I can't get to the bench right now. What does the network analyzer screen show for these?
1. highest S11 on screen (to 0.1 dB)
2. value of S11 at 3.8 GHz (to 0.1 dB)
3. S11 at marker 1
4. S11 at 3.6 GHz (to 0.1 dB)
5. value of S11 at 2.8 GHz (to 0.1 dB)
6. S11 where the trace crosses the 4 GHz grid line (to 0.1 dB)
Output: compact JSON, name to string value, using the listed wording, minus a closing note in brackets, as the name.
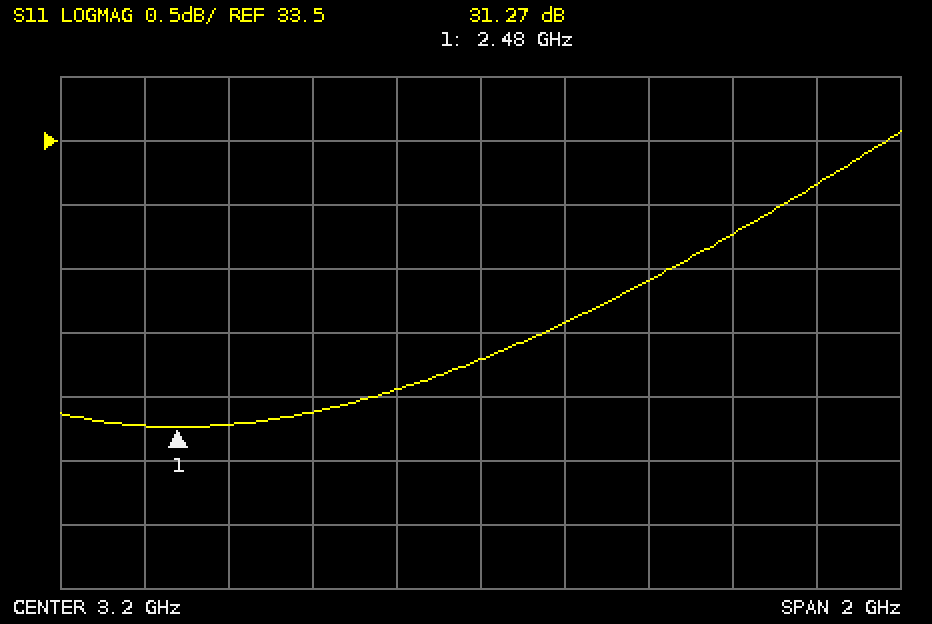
{"highest S11 on screen": "33.6 dB", "value of S11 at 3.8 GHz": "32.8 dB", "S11 at marker 1": "31.27 dB", "S11 at 3.6 GHz": "32.4 dB", "value of S11 at 2.8 GHz": "31.4 dB", "S11 where the trace crosses the 4 GHz grid line": "33.2 dB"}
